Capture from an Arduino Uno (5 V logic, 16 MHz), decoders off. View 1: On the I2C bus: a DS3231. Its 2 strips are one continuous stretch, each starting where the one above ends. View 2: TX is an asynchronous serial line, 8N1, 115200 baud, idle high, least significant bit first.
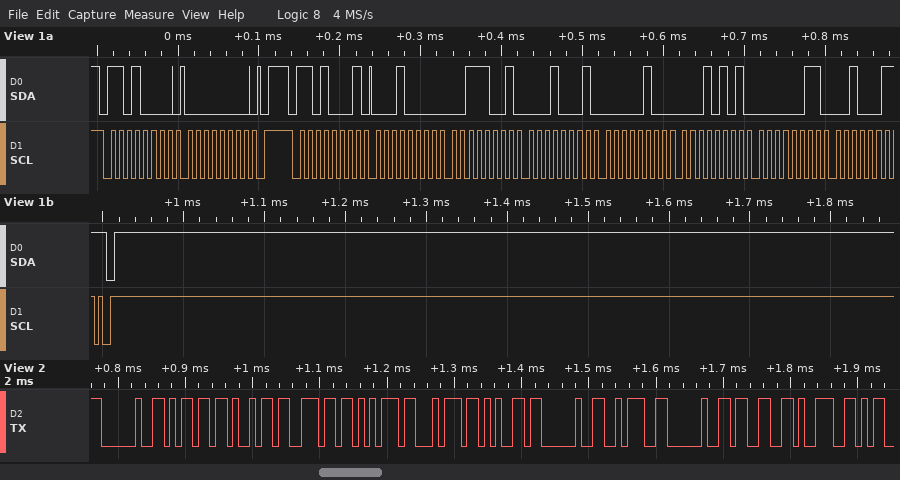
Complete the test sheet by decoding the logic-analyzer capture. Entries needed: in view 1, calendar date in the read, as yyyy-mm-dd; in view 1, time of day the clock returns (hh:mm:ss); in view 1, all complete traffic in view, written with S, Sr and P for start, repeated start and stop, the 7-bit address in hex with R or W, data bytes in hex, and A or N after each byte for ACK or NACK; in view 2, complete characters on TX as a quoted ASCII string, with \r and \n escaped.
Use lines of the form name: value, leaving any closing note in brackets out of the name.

in view 1, calendar date in the read, as yyyy-mm-dd: 2023-03-15
in view 1, time of day the clock returns: 11:39:10
in view 1, all complete traffic in view, written with S, Sr and P for start, repeated start and stop, the 7-bit address in hex with R or W, data bytes in hex, and A or N after each byte for ACK or NACK: S 68W A 00 A P S 68R A 10 A 39 A 11 A 04 A 15 A 03 A 23 N P
in view 2, complete characters on TX as a quoted ASCII string, with \r and \n escaped: " minute : 39"
